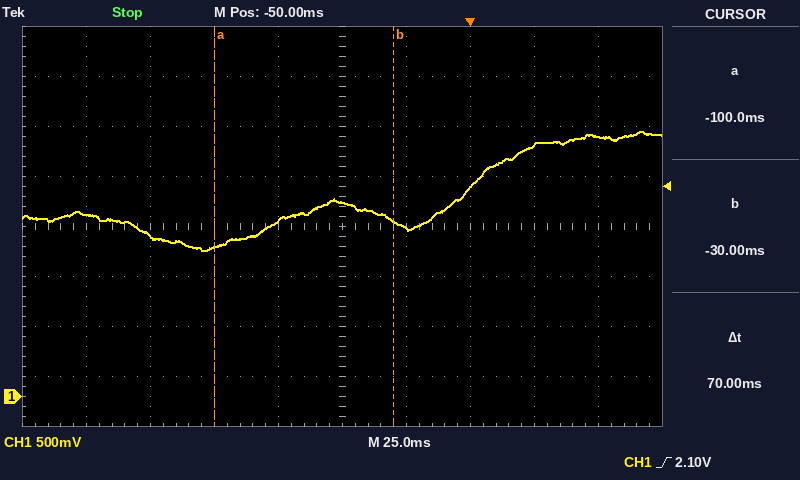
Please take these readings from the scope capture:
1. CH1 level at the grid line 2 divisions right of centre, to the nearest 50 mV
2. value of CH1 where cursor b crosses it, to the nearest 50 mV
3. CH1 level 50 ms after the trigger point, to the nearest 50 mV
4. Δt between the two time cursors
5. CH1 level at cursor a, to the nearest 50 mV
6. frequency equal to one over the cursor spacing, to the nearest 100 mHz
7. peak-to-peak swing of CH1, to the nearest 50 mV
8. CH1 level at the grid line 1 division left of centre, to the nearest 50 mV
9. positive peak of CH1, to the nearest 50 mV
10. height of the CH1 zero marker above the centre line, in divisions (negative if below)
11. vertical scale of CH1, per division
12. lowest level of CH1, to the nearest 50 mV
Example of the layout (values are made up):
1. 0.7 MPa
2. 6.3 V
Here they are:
1. 2.10 V
2. 1.75 V
3. 2.60 V
4. 70 ms
5. 1.50 V
6. 14.3 Hz
7. 1.20 V
8. 1.75 V
9. 2.65 V
10. -3.4 div
11. 500 mV
12. 1.45 V
